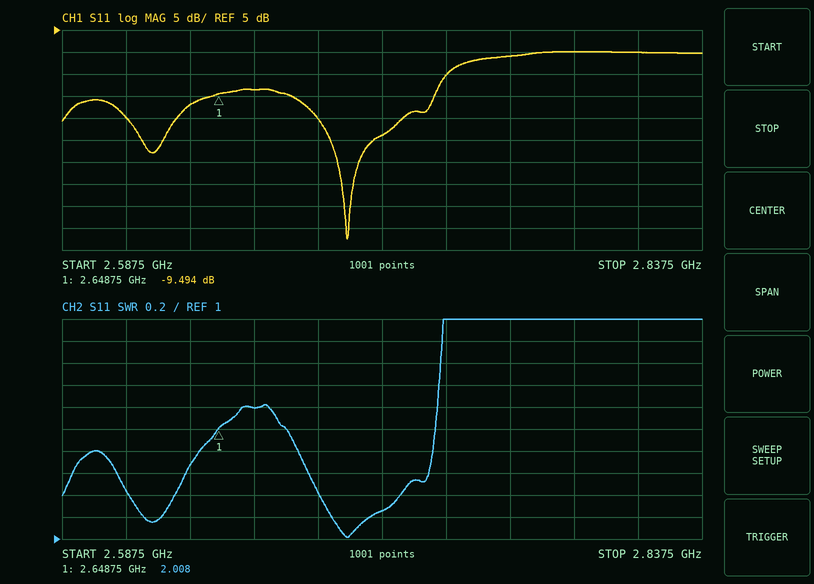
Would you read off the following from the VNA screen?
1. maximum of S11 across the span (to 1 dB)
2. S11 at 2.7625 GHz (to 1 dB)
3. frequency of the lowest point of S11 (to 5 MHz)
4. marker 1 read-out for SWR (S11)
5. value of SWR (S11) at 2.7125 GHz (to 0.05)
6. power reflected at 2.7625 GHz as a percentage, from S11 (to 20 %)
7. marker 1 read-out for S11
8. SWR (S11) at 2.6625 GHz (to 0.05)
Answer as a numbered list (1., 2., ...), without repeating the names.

1. 0 dB
2. -1 dB
3. 2.700 GHz
4. 2.008
5. 1.25
6. 80 %
7. -9.494 dB
8. 2.20
